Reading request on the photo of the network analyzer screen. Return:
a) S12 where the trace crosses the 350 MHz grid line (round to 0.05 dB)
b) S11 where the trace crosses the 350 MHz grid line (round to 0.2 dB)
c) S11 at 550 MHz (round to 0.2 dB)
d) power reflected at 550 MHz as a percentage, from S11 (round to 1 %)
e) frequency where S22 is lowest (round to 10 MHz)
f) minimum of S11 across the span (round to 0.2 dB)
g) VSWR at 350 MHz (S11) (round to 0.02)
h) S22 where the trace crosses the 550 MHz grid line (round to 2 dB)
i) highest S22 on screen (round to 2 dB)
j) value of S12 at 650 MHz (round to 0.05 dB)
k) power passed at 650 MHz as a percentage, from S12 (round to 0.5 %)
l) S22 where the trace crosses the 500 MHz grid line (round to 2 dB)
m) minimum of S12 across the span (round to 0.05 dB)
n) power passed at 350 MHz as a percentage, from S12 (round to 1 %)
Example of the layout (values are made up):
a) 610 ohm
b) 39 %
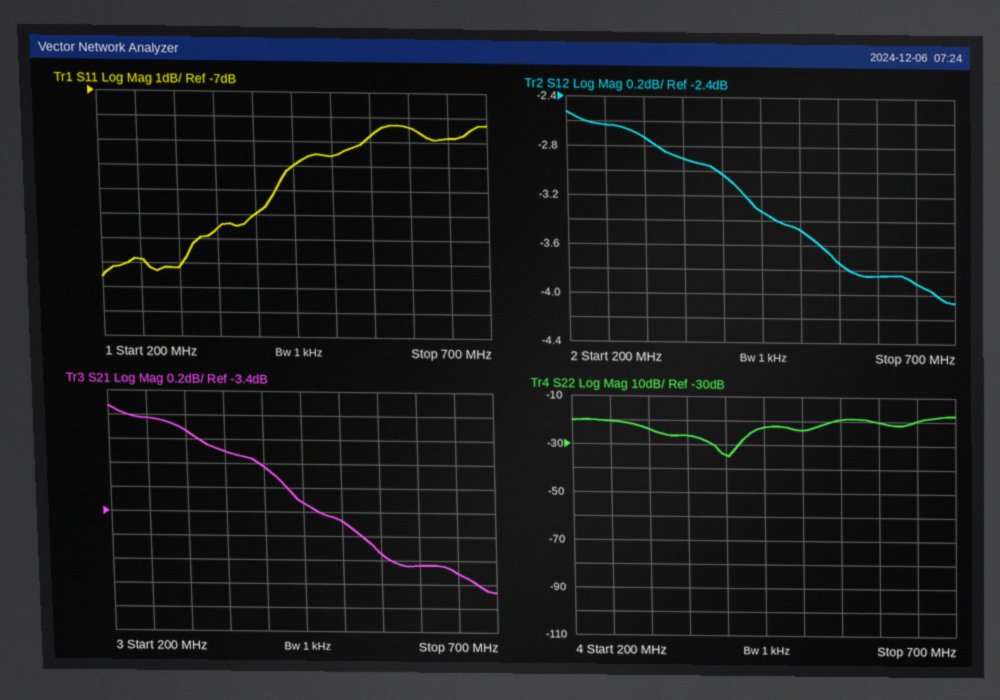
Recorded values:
a) -2.90 dB
b) -12.6 dB
c) -8.8 dB
d) 13 %
e) 400 MHz
f) -14.6 dB
g) 1.62
h) -20 dB
i) -18 dB
j) -3.90 dB
k) 40.5 %
l) -24 dB
m) -4.05 dB
n) 51 %
